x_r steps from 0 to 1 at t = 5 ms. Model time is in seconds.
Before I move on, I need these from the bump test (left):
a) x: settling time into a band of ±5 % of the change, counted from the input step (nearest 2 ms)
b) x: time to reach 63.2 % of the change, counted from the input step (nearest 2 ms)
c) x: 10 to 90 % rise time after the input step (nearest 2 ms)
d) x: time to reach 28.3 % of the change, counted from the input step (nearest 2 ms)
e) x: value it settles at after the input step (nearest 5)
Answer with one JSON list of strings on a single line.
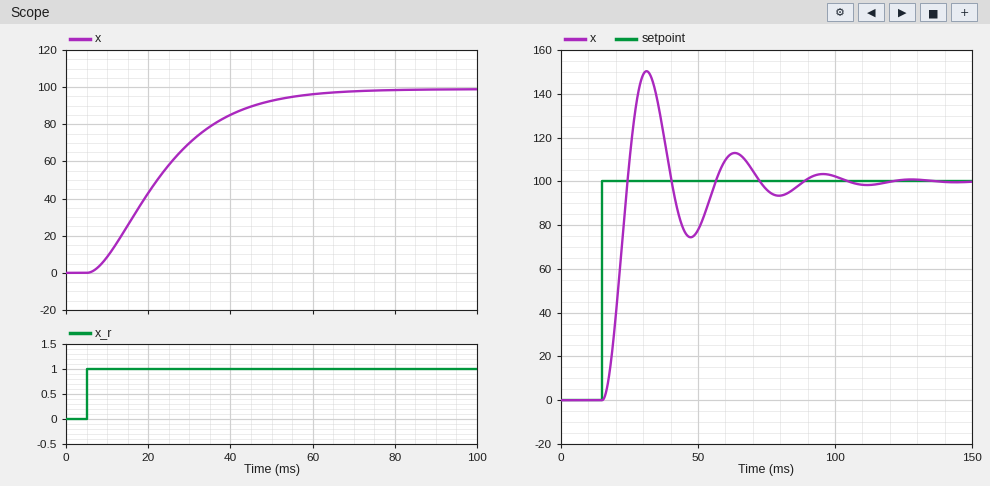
["48 ms", "22 ms", "34 ms", "10 ms", "100"]
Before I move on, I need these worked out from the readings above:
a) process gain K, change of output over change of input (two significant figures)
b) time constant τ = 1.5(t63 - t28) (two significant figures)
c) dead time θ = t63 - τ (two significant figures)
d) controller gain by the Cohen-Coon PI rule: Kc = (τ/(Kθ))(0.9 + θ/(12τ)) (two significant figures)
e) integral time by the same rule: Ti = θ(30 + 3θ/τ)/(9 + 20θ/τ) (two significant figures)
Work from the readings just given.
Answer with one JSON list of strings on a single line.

["100", "18 ms", "4.0 ms", "0.041", "9.1 ms"]
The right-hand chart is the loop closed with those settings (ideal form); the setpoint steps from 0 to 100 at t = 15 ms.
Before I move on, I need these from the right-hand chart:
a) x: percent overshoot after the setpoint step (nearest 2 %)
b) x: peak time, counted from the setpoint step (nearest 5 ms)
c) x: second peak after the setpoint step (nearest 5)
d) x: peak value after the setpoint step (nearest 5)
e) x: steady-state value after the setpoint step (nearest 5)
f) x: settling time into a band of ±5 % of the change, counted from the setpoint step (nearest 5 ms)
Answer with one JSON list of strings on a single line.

["50 %", "15 ms", "115", "150", "100", "70 ms"]
